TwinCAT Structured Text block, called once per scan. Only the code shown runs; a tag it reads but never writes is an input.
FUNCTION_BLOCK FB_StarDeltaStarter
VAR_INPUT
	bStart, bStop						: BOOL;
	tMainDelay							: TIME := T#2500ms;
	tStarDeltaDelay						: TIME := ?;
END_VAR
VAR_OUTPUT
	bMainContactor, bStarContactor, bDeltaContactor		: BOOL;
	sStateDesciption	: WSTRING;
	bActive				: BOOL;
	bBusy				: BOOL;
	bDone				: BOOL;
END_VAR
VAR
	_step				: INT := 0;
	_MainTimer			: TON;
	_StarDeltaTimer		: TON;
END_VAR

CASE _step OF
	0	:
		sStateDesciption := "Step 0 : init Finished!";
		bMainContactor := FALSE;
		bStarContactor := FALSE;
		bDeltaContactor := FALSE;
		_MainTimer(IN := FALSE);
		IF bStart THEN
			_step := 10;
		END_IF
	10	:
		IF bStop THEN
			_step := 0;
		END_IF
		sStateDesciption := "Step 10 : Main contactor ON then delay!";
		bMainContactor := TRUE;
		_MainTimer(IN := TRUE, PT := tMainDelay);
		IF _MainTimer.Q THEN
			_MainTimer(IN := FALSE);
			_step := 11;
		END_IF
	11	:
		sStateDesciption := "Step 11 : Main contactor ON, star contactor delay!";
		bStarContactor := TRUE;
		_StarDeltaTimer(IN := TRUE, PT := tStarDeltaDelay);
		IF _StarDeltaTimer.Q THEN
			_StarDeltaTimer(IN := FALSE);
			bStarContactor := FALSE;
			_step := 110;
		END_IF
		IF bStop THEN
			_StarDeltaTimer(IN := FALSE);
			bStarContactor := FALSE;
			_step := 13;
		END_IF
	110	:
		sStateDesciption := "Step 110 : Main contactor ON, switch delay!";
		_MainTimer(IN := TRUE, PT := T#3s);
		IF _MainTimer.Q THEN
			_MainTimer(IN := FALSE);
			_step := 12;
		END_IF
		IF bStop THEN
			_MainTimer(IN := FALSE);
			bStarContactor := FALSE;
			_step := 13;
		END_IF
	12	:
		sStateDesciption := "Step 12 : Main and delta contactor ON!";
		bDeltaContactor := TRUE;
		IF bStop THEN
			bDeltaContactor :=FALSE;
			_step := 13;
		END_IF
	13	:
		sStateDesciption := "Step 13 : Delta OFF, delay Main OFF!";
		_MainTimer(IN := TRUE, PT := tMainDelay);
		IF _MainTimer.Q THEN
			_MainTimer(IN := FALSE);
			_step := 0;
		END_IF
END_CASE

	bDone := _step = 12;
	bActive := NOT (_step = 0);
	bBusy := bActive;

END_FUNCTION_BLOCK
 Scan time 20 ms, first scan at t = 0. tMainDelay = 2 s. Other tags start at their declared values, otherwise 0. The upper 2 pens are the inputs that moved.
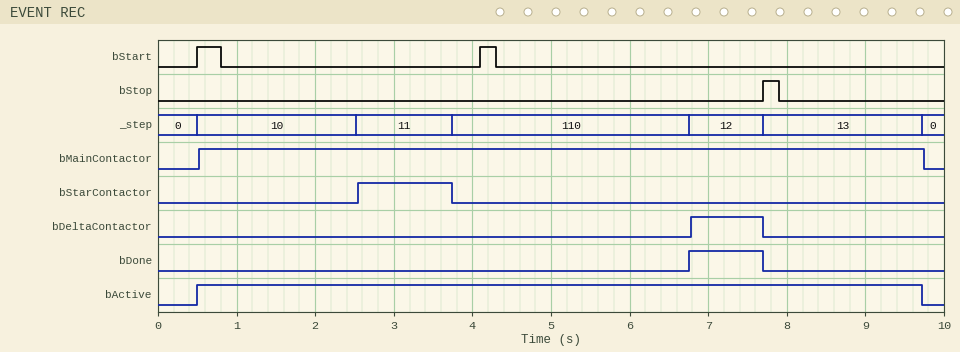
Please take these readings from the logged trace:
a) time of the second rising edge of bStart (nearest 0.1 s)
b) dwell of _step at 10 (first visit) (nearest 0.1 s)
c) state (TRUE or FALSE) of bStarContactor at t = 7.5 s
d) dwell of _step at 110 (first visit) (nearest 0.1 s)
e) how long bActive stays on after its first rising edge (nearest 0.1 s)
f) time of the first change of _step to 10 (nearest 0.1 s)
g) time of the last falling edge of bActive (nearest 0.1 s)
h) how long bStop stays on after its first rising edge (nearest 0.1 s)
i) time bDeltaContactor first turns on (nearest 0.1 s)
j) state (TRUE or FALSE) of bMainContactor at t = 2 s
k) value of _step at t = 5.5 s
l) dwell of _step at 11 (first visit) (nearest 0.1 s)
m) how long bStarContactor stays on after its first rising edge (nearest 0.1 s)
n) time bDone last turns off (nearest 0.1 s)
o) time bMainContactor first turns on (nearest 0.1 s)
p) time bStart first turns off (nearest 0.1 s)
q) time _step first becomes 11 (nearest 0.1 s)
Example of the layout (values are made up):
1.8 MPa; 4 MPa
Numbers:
4.1 s; 2.0 s; FALSE; 3.0 s; 9.2 s; 0.5 s; 9.7 s; 0.2 s; 6.8 s; TRUE; 110; 1.2 s; 1.2 s; 7.7 s; 0.5 s; 0.8 s; 2.5 s
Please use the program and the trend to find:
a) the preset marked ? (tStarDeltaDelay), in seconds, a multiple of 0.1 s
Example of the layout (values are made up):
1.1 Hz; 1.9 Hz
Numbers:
1.2 s
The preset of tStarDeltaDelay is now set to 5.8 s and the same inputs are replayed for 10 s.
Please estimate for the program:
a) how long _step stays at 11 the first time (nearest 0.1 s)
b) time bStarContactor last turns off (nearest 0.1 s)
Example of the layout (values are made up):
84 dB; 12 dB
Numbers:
5.2 s; 7.7 s
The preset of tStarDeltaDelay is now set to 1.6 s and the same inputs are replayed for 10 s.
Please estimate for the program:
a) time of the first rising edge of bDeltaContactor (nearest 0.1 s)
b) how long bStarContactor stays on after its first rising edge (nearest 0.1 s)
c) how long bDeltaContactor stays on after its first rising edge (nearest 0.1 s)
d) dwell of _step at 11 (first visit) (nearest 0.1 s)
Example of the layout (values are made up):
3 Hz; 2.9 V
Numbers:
7.2 s; 1.6 s; 0.5 s; 1.6 s
